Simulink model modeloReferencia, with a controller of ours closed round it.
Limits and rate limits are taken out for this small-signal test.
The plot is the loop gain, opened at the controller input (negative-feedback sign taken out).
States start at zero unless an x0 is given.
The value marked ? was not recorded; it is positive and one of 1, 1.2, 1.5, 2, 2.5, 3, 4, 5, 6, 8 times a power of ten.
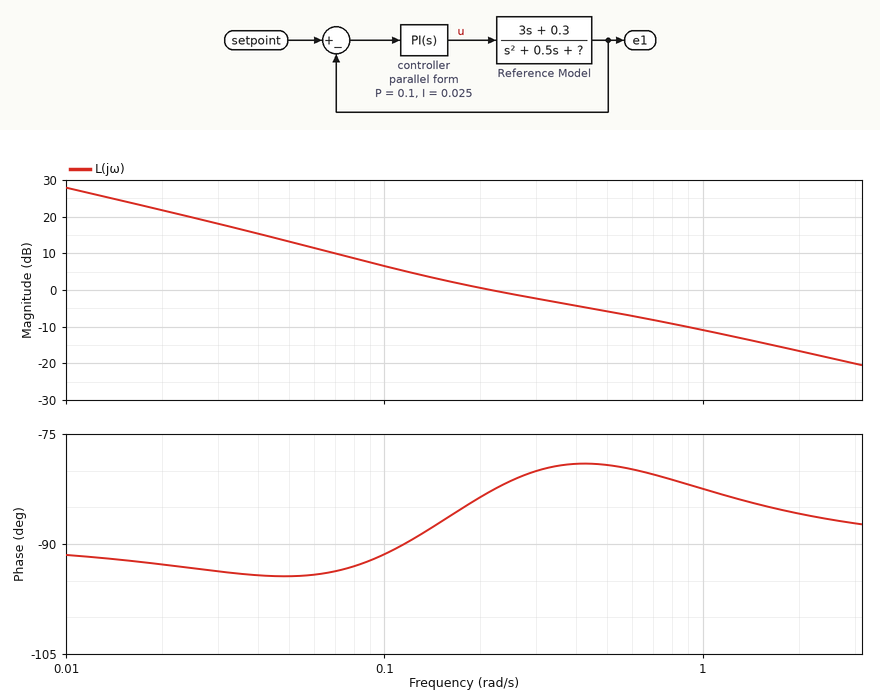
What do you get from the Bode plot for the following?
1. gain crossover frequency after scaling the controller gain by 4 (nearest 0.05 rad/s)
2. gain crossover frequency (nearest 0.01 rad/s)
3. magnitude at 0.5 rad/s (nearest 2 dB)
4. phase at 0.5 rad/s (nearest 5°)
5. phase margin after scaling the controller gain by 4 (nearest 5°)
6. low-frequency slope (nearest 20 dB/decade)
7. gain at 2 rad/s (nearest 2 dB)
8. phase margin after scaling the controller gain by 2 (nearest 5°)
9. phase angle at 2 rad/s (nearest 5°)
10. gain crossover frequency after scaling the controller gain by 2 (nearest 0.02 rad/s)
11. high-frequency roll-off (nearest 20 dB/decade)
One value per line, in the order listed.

1.15 rad/s
0.22 rad/s
-6 dB
-80°
95°
-20 dB/decade
-16 dB
100°
-85°
0.52 rad/s
-20 dB/decade
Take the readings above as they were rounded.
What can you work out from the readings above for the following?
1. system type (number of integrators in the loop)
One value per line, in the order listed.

1
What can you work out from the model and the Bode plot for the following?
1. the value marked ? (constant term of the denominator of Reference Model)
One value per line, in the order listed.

0.03
